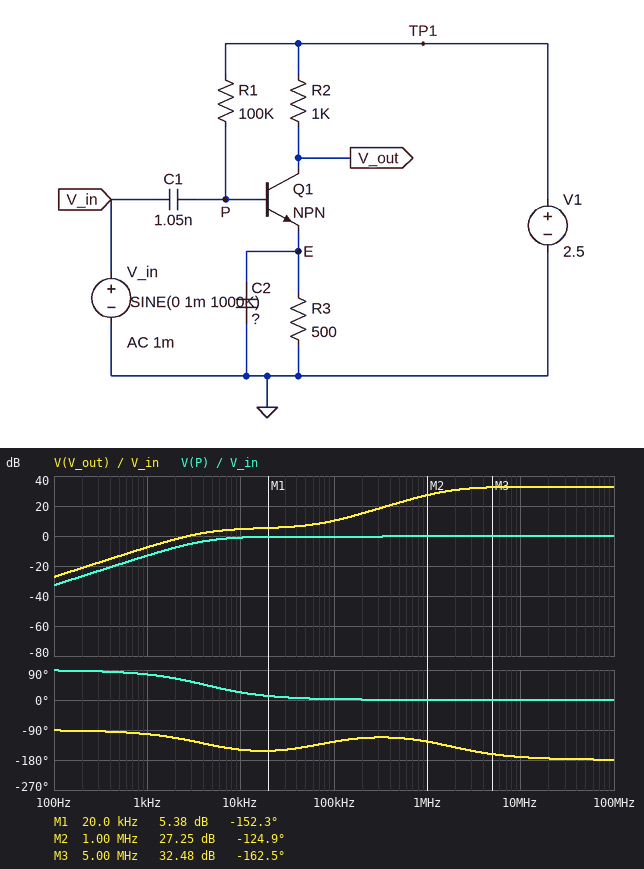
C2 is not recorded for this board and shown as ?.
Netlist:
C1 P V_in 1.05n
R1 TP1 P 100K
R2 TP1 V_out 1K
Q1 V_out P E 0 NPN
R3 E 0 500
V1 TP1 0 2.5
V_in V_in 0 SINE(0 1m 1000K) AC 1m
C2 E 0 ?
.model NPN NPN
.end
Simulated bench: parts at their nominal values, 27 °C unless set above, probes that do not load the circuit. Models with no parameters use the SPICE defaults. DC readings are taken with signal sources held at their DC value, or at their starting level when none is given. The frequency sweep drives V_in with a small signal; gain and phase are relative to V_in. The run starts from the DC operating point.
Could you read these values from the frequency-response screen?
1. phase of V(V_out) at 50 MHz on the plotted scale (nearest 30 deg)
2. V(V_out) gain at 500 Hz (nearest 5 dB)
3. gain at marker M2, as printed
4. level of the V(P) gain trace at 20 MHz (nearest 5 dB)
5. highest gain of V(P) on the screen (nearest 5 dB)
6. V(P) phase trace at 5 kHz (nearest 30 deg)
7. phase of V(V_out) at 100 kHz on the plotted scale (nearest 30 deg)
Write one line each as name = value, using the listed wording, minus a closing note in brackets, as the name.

phase of V(V_out) at 50 MHz on the plotted scale = -180 deg
V(V_out) gain at 500 Hz = -15 dB
gain at marker M2, as printed = 27.25 dB
level of the V(P) gain trace at 20 MHz = 0 dB
highest gain of V(P) on the screen = 0 dB
V(P) phase trace at 5 kHz = 30 deg
phase of V(V_out) at 100 kHz on the plotted scale = -120 deg
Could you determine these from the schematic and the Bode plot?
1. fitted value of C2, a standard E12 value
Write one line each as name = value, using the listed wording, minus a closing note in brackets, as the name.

fitted value of C2, a standard E12 value = 4.7 nF
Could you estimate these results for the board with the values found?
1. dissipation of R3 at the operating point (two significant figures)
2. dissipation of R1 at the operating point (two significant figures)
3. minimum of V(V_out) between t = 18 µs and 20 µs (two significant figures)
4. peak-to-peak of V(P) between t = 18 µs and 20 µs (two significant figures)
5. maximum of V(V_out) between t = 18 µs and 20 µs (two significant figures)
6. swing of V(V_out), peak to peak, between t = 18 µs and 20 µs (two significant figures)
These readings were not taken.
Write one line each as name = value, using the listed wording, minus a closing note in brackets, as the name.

dissipation of R3 at the operating point = 670 µW
dissipation of R1 at the operating point = 13 µW
minimum of V(V_out) between t = 18 µs and 20 µs = 1.3 V
peak-to-peak of V(P) between t = 18 µs and 20 µs = 1.9 mV
maximum of V(V_out) between t = 18 µs and 20 µs = 1.4 V
swing of V(V_out), peak to peak, between t = 18 µs and 20 µs = 46 mV
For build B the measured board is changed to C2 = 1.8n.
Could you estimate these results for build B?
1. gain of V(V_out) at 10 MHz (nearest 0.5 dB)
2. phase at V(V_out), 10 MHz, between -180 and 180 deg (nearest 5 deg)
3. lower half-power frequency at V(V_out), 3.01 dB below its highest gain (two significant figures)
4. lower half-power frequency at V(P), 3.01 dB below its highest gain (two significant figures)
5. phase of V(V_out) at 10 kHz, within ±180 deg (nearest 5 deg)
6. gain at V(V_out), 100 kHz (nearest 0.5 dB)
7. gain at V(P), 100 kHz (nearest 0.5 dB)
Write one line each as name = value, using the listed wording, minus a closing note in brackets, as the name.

gain of V(V_out) at 10 MHz = 32.0 dB
phase at V(V_out), 10 MHz, between -180 and 180 deg = -160 deg
lower half-power frequency at V(V_out), 3.01 dB below its highest gain = 4.2 MHz
lower half-power frequency at V(P), 3.01 dB below its highest gain = 4.5 kHz
phase of V(V_out) at 10 kHz, within ±180 deg = -155 deg
gain at V(V_out), 100 kHz = 6.5 dB
gain at V(P), 100 kHz = 0 dB
